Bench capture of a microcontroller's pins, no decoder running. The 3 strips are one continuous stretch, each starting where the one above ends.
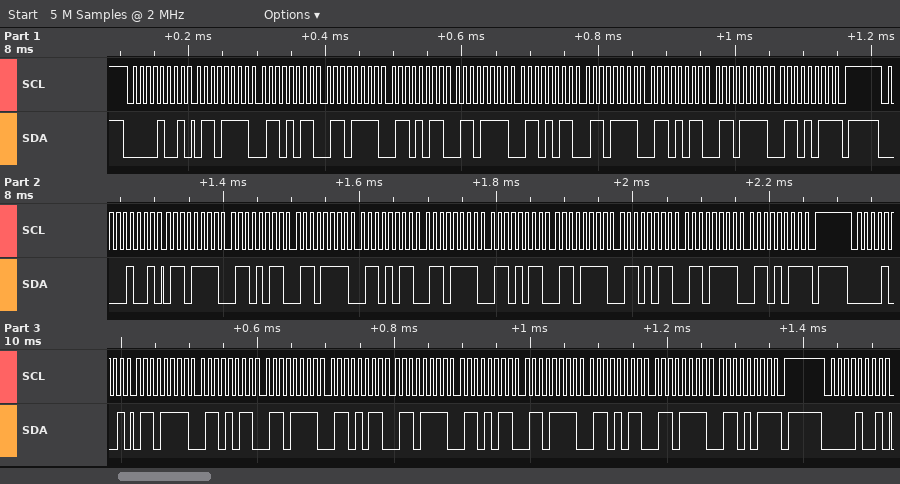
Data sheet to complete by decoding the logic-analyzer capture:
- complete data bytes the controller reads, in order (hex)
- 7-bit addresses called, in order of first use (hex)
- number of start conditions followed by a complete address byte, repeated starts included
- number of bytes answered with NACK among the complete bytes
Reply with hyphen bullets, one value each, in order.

- 6F 6B 6F 6B 6F 6B 6F 6B 6F 6B 6F 6B 6F 6B 6F 6B 6F 6B 6F 6B 6F 6B 6F 6B 6F 6B 6F 6B 6F 6B
- 0x04
- 4
- 3
